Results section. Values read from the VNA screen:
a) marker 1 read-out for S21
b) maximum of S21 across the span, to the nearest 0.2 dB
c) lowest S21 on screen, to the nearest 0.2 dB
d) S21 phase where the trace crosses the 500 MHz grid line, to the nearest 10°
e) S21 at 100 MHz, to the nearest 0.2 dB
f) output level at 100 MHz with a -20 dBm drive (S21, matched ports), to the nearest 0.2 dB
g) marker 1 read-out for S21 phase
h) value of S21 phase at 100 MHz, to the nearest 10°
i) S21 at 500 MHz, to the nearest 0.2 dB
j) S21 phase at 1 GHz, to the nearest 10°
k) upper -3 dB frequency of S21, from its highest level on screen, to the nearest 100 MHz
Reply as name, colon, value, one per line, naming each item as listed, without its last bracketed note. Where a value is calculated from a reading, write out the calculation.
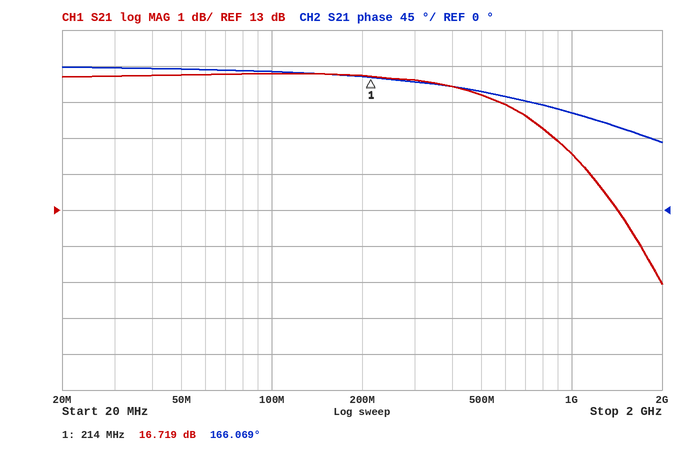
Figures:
marker 1 read-out for S21: 16.719 dB
maximum of S21 across the span, to the nearest 0.2 dB: 16.8 dB
lowest S21 on screen, to the nearest 0.2 dB: 11.0 dB
S21 phase where the trace crosses the 500 MHz grid line, to the nearest 10°: 150°
S21 at 100 MHz, to the nearest 0.2 dB: 16.8 dB
output level at 100 MHz with a -20 dBm drive (S21, matched ports), to the nearest 0.2 dB: -20 dBm + (16.8 dB) = -3.2 dBm
marker 1 read-out for S21 phase: 166.069°
value of S21 phase at 100 MHz, to the nearest 10°: 170°
S21 at 500 MHz, to the nearest 0.2 dB: 16.2 dB
S21 phase at 1 GHz, to the nearest 10°: 120°
upper -3 dB frequency of S21, from its highest level on screen, to the nearest 100 MHz: 1.2 GHz
